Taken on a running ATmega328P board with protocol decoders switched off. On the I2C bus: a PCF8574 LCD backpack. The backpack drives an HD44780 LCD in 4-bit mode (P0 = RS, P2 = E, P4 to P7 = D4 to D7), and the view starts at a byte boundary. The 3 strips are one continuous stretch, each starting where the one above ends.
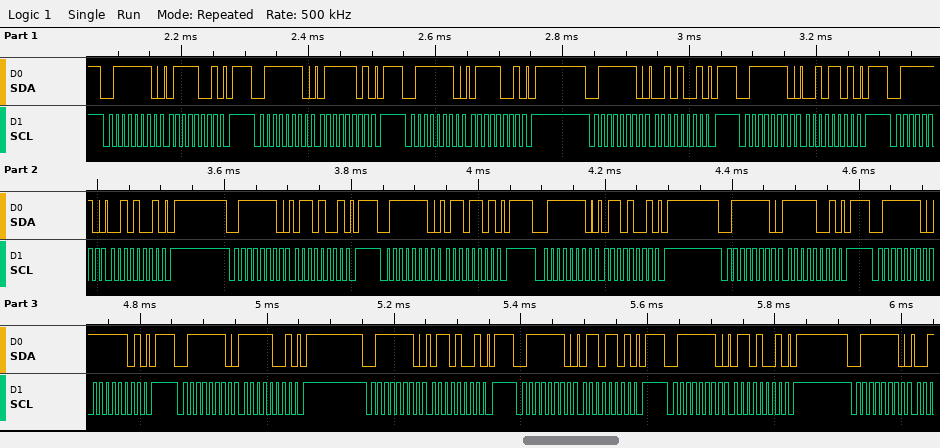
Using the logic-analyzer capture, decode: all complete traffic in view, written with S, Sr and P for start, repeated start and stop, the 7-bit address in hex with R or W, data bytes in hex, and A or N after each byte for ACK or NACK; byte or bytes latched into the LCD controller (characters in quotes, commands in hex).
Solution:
S 3FW A 79 A P S 3FW A 7D A P S 3FW A 79 A P S 3FW A 29 A P S 3FW A 2D A P S 3FW A 29 A P S 3FW A 69 A P S 3FW A 6D A P S 3FW A 69 A P S 3FW A F9 A P S 3FW A FD A P S 3FW A F9 A P S 3FW A 69 A P S 3FW A 6D A P S 3FW A 69 A P S 3FW A
'r' 'o'
